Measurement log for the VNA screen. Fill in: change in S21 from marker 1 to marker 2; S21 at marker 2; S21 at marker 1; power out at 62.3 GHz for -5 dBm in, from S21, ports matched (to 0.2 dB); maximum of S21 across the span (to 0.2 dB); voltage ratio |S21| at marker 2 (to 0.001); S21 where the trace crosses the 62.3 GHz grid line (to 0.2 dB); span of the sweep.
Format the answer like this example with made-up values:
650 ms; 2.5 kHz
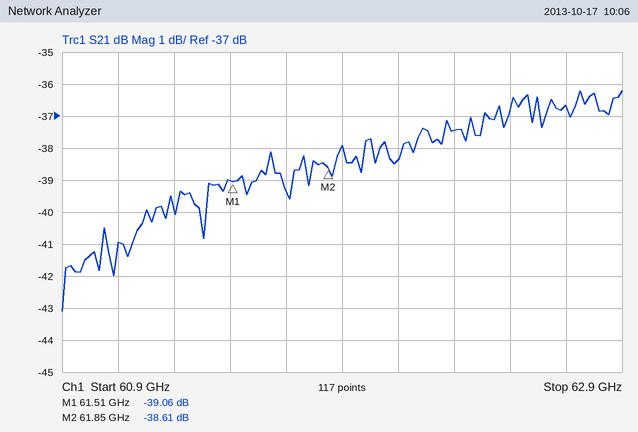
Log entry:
0.45 dB; -38.61 dB; -39.06 dB; -42.4 dBm; -36.2 dB; 0.012; -37.4 dB; 2 GHz
